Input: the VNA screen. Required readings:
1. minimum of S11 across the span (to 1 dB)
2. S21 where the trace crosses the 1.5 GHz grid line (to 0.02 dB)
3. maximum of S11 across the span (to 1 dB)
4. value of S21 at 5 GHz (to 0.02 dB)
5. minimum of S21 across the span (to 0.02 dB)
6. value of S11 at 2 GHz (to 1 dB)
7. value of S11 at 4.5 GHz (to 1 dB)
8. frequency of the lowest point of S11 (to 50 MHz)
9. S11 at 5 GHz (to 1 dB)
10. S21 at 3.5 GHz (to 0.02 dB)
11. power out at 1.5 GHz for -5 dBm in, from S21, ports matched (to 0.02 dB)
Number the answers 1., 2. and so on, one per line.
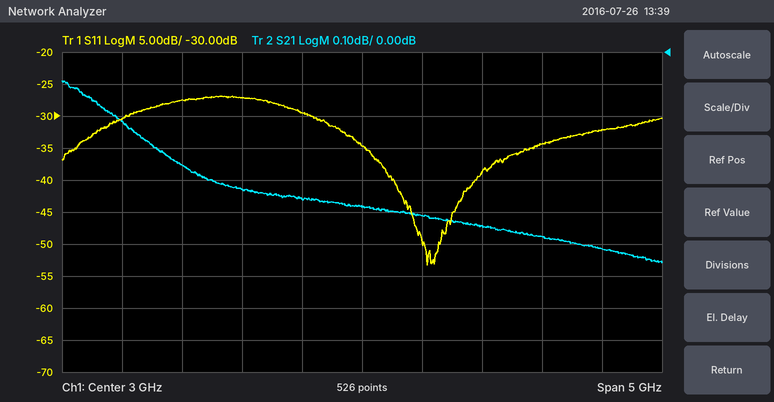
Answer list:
1. -53 dB
2. -0.36 dB
3. -27 dB
4. -0.62 dB
5. -0.66 dB
6. -27 dB
7. -34 dB
8. 3.55 GHz
9. -32 dB
10. -0.52 dB
11. -5.36 dBm
